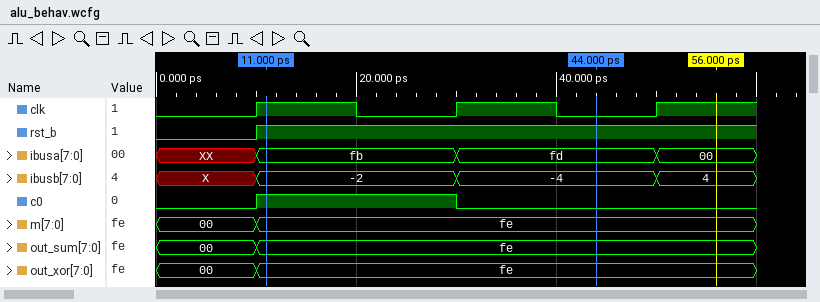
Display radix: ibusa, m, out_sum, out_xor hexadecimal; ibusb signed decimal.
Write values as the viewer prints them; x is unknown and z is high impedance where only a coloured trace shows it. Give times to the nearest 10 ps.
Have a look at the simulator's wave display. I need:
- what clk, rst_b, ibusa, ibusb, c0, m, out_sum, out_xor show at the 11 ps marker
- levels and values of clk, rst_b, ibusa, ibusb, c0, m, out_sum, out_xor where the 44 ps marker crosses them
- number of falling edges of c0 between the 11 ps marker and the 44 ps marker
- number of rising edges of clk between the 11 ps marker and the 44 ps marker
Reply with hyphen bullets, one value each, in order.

- clk=1, rst_b=1, ibusa=fb, ibusb=-2, c0=1, m=fe, out_sum=fe, out_xor=fe
- clk=0, rst_b=1, ibusa=fd, ibusb=-4, c0=0, m=fe, out_sum=fe, out_xor=fe
- 1
- 1
